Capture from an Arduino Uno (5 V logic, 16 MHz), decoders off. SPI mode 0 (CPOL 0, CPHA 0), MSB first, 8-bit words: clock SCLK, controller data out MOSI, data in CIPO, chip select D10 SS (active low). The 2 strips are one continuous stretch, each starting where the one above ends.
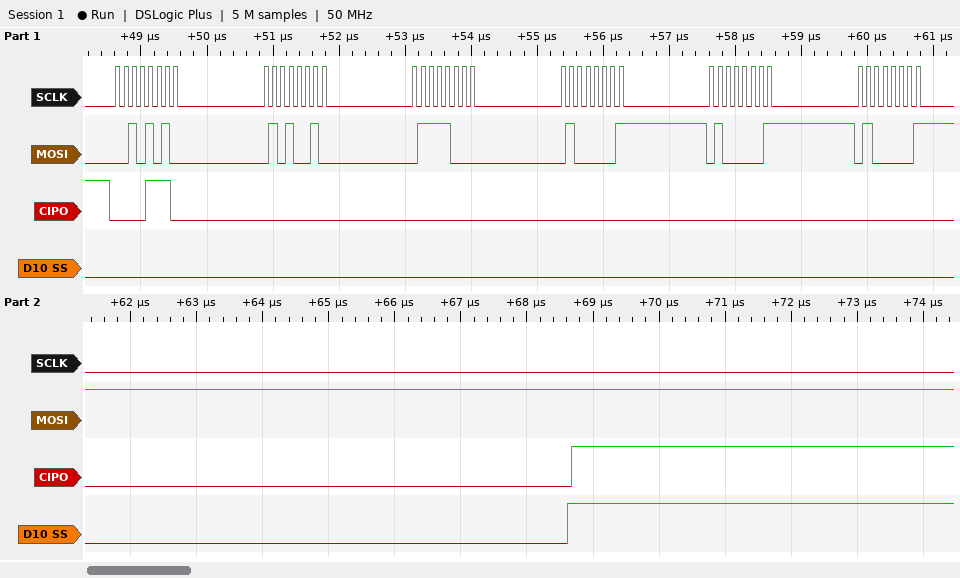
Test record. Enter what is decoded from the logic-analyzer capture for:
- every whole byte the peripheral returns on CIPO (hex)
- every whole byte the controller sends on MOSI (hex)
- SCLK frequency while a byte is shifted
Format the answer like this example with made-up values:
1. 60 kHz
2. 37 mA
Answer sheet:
1. 0E 00 00 00 00 00
2. 2A 52 78 41 41 41
3. 8 MHz
